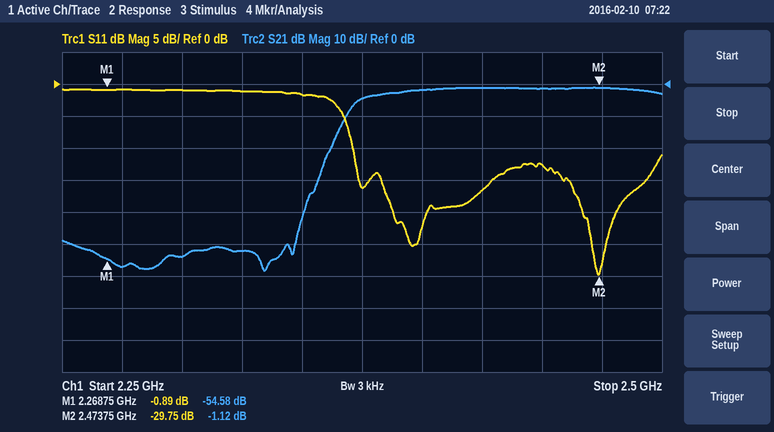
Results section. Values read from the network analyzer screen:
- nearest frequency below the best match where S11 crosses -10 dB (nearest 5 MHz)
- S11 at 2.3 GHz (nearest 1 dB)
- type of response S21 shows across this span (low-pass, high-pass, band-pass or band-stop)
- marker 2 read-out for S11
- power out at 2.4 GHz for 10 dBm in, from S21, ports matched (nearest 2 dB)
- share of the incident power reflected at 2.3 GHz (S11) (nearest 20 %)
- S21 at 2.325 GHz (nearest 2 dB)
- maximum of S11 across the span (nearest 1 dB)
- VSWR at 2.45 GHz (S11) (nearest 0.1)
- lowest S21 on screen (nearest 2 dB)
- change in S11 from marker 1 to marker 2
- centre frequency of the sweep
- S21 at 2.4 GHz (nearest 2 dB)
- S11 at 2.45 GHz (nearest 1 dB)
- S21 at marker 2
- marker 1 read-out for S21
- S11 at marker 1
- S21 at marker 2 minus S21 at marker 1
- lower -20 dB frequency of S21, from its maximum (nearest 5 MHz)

2.370 GHz
-1 dB
high-pass
-29.75 dB
8 dBm
80 %
-52 dB
-1 dB
1.6
-58 dB
-28.86 dB
2.375 GHz
-2 dB
-13 dB
-1.12 dB
-54.58 dB
-0.89 dB
53.46 dB
2.360 GHz
